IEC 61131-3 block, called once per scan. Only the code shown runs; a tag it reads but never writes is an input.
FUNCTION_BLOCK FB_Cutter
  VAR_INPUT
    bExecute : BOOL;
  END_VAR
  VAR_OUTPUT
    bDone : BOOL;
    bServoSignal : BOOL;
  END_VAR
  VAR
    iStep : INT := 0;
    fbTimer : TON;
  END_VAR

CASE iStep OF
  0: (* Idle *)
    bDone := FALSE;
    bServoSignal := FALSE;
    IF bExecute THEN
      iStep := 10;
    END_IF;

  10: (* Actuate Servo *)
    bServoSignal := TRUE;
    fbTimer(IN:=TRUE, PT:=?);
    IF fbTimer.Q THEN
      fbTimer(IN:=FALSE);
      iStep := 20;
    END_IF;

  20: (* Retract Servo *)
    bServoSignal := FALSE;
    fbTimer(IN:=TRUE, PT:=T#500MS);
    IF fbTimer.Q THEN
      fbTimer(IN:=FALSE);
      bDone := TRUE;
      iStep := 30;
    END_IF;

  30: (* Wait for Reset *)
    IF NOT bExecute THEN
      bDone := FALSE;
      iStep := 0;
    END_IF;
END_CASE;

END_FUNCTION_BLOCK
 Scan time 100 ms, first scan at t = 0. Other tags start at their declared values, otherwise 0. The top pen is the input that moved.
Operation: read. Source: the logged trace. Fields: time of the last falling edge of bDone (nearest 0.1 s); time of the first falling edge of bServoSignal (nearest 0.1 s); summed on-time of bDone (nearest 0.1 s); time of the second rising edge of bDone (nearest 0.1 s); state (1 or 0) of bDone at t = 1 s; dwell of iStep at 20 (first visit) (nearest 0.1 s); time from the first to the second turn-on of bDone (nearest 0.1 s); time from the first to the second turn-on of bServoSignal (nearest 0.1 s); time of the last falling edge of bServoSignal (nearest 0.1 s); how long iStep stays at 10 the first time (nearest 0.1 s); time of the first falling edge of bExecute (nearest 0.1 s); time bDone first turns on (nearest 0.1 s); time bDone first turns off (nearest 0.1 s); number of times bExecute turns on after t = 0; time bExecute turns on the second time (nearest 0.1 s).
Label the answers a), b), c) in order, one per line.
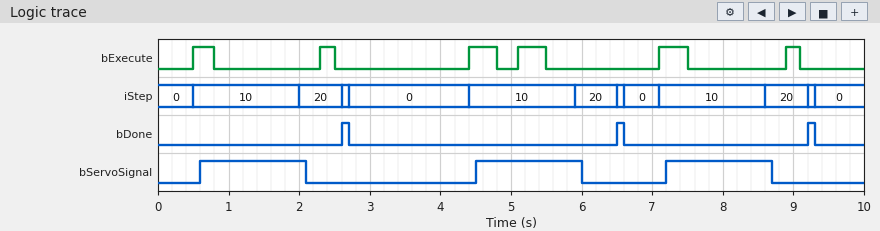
a) 9.3 s
b) 2.1 s
c) 0.3 s
d) 6.5 s
e) 0
f) 0.6 s
g) 3.9 s
h) 3.9 s
i) 8.7 s
j) 1.5 s
k) 0.8 s
l) 2.6 s
m) 2.7 s
n) 6
o) 2.3 s
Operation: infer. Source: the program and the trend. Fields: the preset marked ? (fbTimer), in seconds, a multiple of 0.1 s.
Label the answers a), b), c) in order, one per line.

a) 1.4 s
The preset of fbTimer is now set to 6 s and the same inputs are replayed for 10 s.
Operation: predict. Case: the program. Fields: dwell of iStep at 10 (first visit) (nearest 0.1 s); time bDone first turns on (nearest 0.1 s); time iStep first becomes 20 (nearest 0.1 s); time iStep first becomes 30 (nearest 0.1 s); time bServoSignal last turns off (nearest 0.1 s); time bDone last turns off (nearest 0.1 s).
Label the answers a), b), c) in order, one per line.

a) 6.1 s
b) 7.2 s
c) 6.6 s
d) 7.2 s
e) 6.7 s
f) 7.5 s
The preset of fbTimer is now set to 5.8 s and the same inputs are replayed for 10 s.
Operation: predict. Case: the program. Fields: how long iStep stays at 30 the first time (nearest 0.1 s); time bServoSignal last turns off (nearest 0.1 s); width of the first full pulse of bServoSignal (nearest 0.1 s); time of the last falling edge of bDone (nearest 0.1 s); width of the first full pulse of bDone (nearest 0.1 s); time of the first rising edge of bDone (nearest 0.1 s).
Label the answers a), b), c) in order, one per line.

a) 0.5 s
b) 6.5 s
c) 5.9 s
d) 7.5 s
e) 0.5 s
f) 7.0 s
